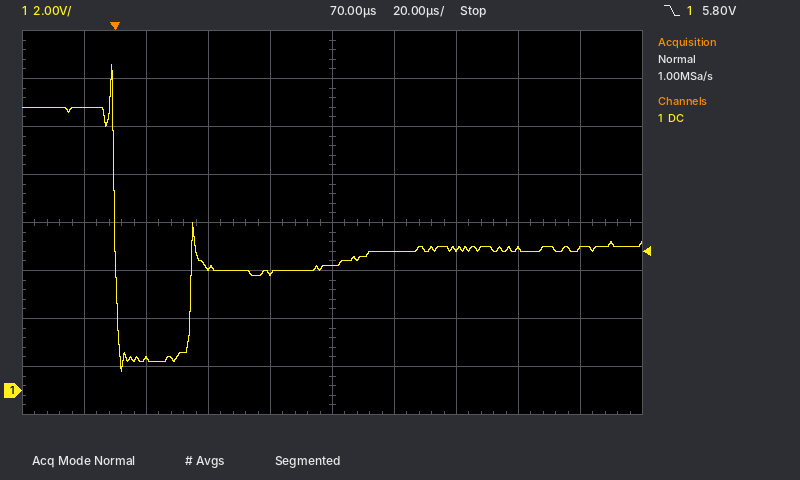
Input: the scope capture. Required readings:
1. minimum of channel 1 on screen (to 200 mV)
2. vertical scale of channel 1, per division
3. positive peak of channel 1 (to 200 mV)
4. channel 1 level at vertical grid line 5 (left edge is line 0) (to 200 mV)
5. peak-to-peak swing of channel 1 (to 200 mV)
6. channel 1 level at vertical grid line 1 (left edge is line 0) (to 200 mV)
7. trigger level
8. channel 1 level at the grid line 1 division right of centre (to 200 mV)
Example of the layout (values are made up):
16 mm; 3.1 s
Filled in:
800 mV; 2 V; 13.6 V; 5.2 V; 12.8 V; 11.8 V; 5.80 V; 5.8 V
